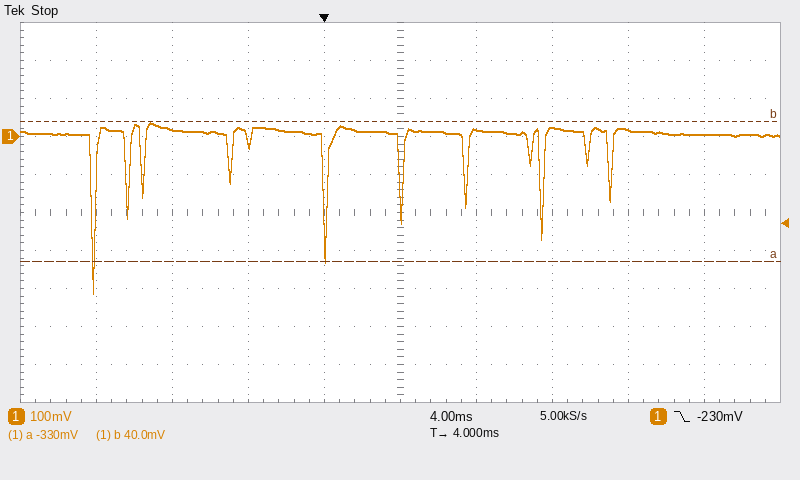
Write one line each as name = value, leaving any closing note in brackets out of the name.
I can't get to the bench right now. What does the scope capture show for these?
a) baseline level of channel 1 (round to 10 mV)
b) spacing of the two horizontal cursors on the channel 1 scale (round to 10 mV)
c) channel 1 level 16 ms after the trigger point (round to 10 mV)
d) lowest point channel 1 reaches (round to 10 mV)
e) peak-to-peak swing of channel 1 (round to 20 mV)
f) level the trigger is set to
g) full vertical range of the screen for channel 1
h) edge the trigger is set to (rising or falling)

baseline level of channel 1 = 10 mV
spacing of the two horizontal cursors on the channel 1 scale = 370 mV
channel 1 level 16 ms after the trigger point = 20 mV
lowest point channel 1 reaches = -410 mV
peak-to-peak swing of channel 1 = 440 mV
level the trigger is set to = -230 mV
full vertical range of the screen for channel 1 = 1 V
edge the trigger is set to = falling
